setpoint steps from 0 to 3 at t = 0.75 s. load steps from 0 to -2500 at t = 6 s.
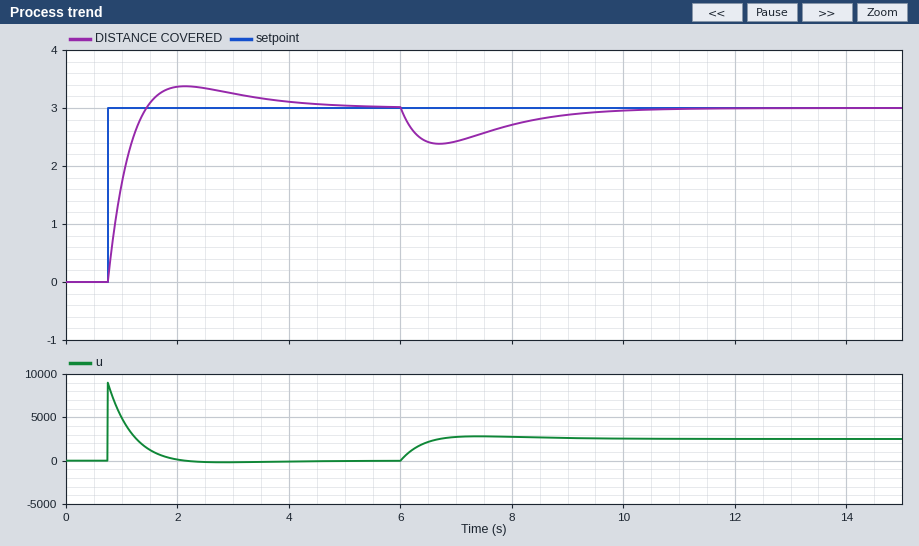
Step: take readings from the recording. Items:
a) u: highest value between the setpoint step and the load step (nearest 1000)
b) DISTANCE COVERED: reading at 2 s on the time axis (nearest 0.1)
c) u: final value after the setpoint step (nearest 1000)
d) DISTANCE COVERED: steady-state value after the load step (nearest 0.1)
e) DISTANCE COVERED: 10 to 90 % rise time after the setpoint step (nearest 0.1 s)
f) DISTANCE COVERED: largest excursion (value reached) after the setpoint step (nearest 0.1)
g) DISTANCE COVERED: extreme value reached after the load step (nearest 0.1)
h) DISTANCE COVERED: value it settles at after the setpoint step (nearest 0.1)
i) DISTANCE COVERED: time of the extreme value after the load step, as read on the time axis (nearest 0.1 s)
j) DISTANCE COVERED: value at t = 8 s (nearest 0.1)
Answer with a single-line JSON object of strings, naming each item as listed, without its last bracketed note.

{"u: highest value between the setpoint step and the load step": "9000", "DISTANCE COVERED: reading at 2 s on the time axis": "3.4", "u: final value after the setpoint step": "0", "DISTANCE COVERED: steady-state value after the load step": "3.0", "DISTANCE COVERED: 10 to 90 % rise time after the setpoint step": "0.5 s", "DISTANCE COVERED: largest excursion (value reached) after the setpoint step": "3.4", "DISTANCE COVERED: extreme value reached after the load step": "2.4", "DISTANCE COVERED: value it settles at after the setpoint step": "3.0", "DISTANCE COVERED: time of the extreme value after the load step, as read on the time axis": "6.7 s", "DISTANCE COVERED: value at t = 8 s": "2.7"}
